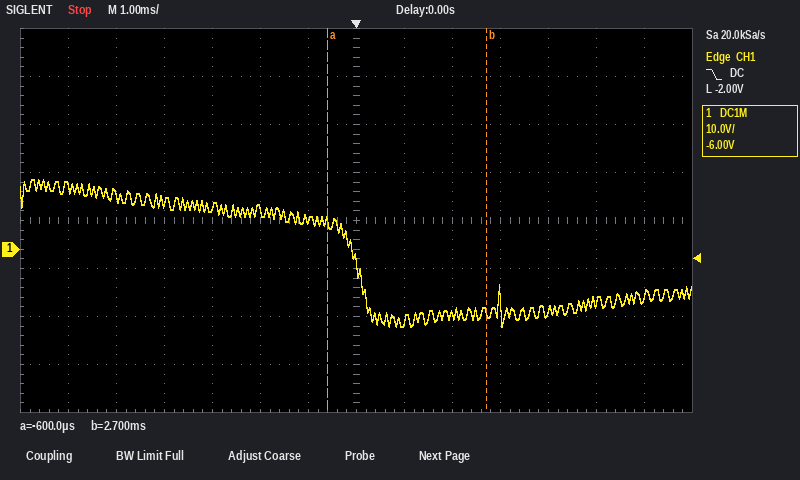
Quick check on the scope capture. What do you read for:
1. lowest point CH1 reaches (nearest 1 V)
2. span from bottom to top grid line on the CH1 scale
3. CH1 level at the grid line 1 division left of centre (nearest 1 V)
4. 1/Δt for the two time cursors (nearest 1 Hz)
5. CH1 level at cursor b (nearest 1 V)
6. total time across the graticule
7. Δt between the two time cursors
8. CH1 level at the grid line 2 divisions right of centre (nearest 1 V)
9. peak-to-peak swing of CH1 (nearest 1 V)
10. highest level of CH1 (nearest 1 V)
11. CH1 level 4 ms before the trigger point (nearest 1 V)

-16 V
80 V
6 V
303 Hz
-13 V
14 ms
3.3 ms
-14 V
31 V
15 V
10 V
